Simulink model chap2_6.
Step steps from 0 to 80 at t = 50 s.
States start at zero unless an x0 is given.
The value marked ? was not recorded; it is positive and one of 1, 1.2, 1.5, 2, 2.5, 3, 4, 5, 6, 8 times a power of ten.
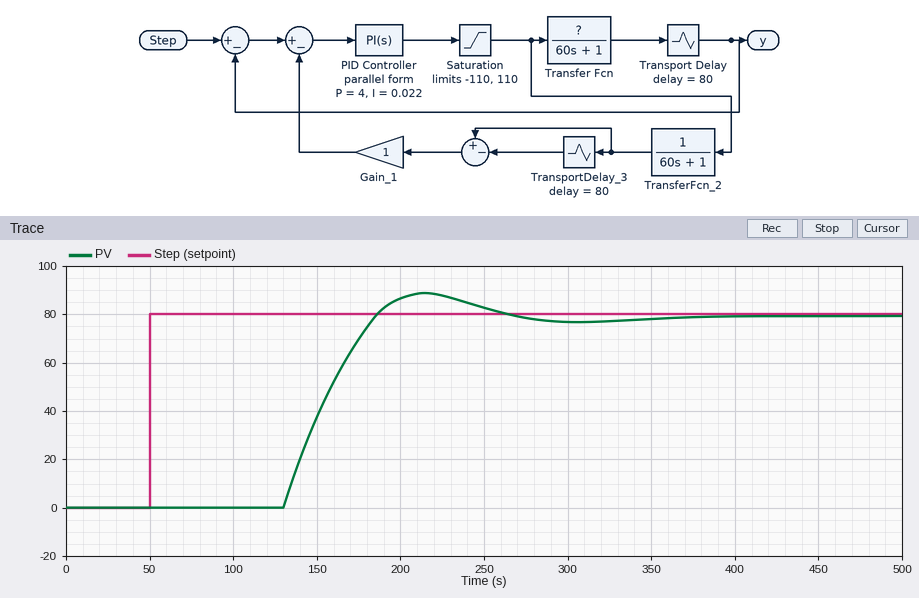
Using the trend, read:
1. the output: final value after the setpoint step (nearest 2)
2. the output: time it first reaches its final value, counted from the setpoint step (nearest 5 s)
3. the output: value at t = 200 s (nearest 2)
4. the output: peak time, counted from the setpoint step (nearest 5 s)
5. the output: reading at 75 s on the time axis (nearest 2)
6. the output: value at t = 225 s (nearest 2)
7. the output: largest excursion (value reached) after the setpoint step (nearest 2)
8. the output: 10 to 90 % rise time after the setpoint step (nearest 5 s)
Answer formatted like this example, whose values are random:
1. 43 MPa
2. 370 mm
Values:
1. 80
2. 135 s
3. 86
4. 165 s
5. 0
6. 88
7. 88
8. 45 s
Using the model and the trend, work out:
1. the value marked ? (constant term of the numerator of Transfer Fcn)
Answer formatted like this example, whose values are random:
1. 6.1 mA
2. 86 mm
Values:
1. 1.2
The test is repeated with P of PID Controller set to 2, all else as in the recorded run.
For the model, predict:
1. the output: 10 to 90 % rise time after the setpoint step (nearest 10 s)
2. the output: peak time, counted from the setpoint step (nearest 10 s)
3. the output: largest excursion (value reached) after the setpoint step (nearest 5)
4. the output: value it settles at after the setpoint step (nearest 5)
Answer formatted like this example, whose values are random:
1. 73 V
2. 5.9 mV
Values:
1. 50 s
2. 180 s
3. 85
4. 80
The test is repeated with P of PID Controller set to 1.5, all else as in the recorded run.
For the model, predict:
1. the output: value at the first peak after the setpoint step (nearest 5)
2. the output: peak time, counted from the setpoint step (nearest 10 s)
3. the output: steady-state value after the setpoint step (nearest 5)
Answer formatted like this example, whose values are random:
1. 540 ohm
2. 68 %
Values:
1. 85
2. 190 s
3. 80
